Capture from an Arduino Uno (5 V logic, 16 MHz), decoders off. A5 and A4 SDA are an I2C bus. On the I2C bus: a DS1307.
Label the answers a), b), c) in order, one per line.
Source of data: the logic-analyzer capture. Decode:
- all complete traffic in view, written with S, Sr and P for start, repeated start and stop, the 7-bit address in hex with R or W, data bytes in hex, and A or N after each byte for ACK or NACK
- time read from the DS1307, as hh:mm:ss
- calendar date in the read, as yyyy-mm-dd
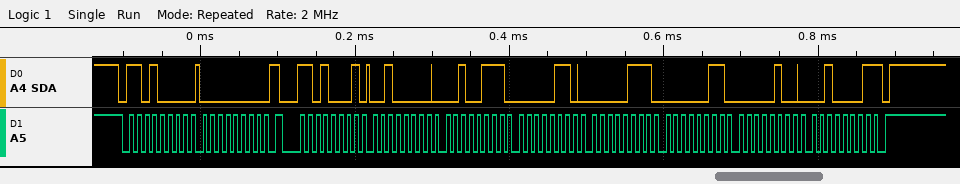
a) S 68W A 00 A Sr 68R A 20 A 27 A 06 A 07 A 03 A 04 A 21 N P
b) 06:27:20
c) 2021-04-03
